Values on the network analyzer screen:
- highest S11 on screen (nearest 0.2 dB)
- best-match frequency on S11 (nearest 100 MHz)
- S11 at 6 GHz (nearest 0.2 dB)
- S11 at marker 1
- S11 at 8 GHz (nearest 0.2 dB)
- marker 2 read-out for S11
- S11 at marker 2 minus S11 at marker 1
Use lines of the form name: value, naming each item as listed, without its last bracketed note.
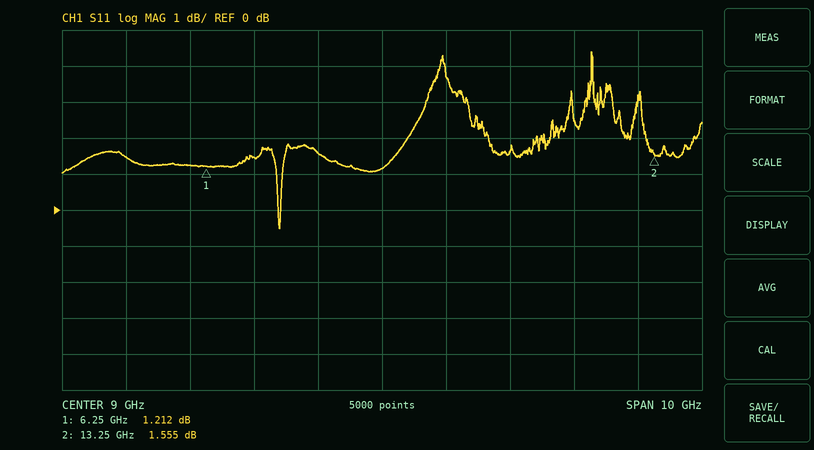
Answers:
highest S11 on screen: 4.4 dB
best-match frequency on S11: 7.4 GHz
S11 at 6 GHz: 1.2 dB
S11 at marker 1: 1.212 dB
S11 at 8 GHz: 1.6 dB
marker 2 read-out for S11: 1.555 dB
S11 at marker 2 minus S11 at marker 1: 0.343 dB
